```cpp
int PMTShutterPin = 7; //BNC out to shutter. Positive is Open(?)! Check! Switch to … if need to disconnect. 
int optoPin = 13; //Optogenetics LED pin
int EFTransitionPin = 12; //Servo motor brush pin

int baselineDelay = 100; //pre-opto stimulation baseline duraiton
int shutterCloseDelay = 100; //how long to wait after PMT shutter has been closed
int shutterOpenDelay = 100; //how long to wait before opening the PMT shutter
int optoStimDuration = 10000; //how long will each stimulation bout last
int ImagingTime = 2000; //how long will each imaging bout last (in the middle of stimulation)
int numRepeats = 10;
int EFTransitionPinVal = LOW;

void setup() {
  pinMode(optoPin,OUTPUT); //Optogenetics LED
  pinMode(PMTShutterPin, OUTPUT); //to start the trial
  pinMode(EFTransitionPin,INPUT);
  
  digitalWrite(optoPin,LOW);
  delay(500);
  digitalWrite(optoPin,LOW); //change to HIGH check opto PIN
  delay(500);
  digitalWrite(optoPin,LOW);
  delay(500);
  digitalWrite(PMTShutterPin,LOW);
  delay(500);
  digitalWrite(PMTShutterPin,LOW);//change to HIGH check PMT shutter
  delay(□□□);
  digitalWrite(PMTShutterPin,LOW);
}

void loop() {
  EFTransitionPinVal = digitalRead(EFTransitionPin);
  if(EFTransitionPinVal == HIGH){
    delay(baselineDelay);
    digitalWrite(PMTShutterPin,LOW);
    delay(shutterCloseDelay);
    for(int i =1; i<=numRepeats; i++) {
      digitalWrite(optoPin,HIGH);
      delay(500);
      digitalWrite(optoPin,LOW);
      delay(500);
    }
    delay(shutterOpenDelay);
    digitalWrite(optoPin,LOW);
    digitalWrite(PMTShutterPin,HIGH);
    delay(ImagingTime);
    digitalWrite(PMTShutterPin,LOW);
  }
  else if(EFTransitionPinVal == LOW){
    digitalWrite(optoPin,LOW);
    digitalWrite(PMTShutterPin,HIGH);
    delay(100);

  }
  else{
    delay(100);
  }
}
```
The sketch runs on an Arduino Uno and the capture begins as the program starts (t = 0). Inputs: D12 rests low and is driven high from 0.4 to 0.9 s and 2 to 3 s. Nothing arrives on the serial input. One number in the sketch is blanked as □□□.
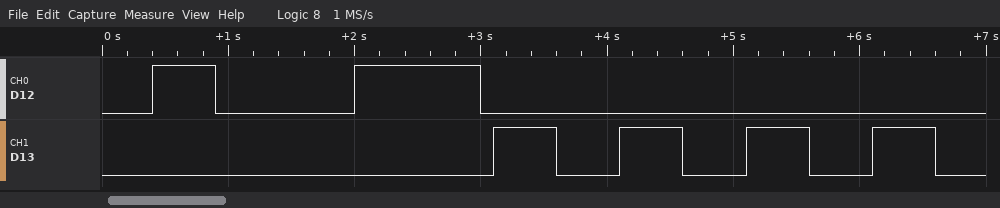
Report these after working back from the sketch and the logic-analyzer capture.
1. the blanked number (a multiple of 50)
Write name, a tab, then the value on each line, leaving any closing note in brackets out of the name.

the blanked number	900
